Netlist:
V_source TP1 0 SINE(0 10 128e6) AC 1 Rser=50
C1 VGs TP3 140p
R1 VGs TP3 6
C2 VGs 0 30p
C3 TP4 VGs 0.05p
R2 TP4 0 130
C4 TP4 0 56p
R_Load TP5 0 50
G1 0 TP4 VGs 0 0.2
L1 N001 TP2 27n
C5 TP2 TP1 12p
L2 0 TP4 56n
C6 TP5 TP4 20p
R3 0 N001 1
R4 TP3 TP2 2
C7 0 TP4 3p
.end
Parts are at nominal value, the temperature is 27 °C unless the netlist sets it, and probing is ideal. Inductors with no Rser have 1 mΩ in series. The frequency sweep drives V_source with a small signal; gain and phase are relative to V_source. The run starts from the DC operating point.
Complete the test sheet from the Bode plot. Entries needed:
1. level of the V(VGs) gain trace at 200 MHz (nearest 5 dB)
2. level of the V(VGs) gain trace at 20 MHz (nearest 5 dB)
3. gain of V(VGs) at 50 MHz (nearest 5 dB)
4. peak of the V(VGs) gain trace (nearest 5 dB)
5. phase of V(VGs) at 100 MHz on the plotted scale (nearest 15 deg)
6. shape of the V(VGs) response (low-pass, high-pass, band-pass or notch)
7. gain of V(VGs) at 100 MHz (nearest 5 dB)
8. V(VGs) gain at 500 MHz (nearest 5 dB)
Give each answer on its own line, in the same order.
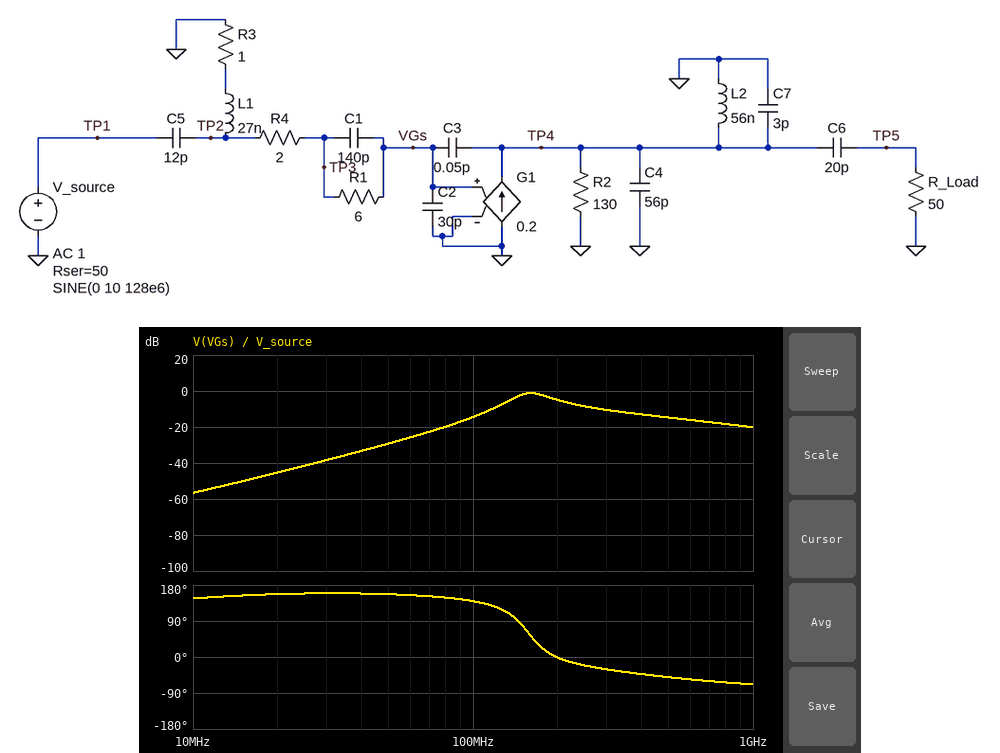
-5 dB
-45 dB
-30 dB
0 dB
135 deg
band-pass
-15 dB
-15 dB
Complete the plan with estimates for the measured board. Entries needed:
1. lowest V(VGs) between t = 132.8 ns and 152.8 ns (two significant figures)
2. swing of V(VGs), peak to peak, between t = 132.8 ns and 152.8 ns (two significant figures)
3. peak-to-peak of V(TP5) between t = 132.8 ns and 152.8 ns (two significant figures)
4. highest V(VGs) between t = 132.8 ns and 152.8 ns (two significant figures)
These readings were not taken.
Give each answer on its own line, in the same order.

-4.4 V
8.9 V
29 V
4.4 V
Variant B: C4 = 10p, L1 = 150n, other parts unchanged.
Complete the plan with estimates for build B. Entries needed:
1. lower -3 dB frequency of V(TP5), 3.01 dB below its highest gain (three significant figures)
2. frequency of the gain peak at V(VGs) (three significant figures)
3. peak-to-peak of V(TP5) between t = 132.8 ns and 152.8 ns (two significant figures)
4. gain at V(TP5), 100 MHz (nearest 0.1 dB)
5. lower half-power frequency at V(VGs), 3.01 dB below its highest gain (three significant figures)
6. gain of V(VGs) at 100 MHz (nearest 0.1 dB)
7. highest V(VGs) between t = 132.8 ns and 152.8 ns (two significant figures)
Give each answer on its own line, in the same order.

61.1 MHz
64.5 MHz
58 V
9.1 dB
59.9 MHz
-6.6 dB
3.6 V
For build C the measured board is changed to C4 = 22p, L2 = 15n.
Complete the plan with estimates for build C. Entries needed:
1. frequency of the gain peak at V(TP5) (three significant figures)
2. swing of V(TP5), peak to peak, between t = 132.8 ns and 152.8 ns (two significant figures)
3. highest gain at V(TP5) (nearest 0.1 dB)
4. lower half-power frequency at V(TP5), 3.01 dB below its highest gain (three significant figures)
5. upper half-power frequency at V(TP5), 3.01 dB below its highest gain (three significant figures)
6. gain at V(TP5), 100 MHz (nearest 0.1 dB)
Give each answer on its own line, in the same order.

188 MHz
20 V
11.8 dB
152 MHz
253 MHz
-12.2 dB
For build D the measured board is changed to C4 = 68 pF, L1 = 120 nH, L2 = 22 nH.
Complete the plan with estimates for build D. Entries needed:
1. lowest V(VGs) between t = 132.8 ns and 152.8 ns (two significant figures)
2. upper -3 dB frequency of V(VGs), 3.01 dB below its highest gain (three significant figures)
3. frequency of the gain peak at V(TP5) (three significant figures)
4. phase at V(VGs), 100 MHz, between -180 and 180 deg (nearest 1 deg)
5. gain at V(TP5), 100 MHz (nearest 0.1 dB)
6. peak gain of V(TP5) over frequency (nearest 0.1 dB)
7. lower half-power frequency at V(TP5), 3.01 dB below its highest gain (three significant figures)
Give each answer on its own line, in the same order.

-3.9 V
79.4 MHz
115 MHz
-3 deg
8.2 dB
11.1 dB
99.4 MHz
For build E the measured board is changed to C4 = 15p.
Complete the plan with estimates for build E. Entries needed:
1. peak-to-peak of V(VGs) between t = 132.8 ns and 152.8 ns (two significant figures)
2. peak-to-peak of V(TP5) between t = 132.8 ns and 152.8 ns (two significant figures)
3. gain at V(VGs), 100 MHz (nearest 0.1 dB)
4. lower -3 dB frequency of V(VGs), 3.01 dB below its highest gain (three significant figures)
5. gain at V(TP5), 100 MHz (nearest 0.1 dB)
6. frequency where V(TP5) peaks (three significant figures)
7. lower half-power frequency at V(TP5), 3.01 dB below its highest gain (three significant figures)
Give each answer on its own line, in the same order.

8.7 V
70 V
-14.5 dB
140 MHz
2.1 dB
158 MHz
136 MHz
